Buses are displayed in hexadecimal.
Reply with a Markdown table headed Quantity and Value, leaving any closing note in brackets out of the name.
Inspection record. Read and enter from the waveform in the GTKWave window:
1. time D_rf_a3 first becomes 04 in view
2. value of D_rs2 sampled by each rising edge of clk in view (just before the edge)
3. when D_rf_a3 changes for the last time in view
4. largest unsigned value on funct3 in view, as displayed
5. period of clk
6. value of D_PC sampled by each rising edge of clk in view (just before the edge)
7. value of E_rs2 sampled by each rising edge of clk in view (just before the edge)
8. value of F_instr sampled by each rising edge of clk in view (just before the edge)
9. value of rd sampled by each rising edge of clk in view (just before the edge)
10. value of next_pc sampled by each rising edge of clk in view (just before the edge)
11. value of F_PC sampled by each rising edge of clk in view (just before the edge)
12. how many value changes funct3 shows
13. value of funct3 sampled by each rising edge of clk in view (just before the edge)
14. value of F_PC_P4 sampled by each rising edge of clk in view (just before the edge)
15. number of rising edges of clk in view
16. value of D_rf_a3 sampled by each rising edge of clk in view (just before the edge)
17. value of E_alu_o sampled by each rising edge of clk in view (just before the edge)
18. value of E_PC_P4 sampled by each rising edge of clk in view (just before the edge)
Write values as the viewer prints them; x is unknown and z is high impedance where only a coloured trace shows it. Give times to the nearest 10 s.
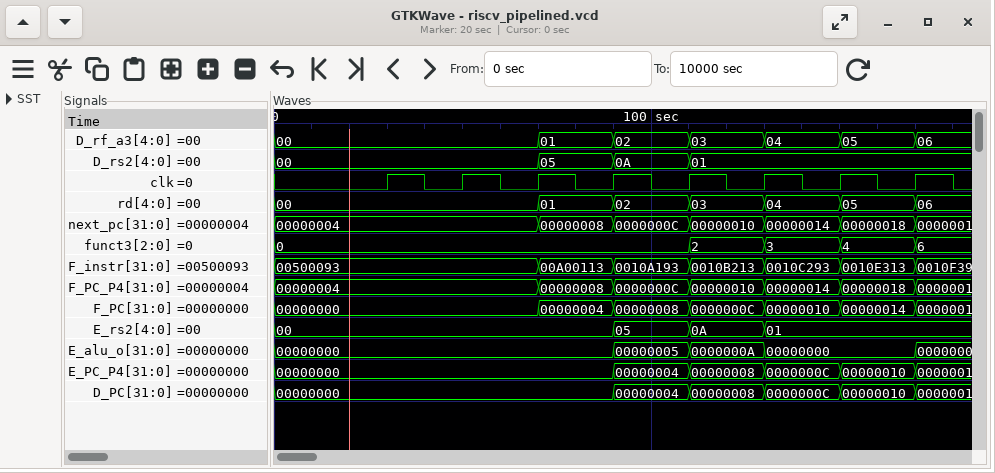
| Quantity | Value |
|---|---|
| time D_rf_a3 first becomes 04 in view | 130 s |
| value of D_rs2 sampled by each rising edge of clk in view | 00, 00, 00, 05, 0A, 01, 01, 01 |
| when D_rf_a3 changes for the last time in view | 170 s |
| largest unsigned value on funct3 in view, as displayed | 6 |
| period of clk | 20 s |
| value of D_PC sampled by each rising edge of clk in view | 00000000, 00000000, 00000000, 00000000, 00000004, 00000008, 0000000C, 00000010 |
| value of E_rs2 sampled by each rising edge of clk in view | 00, 00, 00, 00, 05, 0A, 01, 01 |
| value of F_instr sampled by each rising edge of clk in view | 00500093, 00500093, 00500093, 00A00113, 0010A193, 0010B213, 0010C293, 0010E313 |
| value of rd sampled by each rising edge of clk in view | 00, 00, 00, 01, 02, 03, 04, 05 |
| value of next_pc sampled by each rising edge of clk in view | 00000004, 00000004, 00000004, 00000008, 0000000C, 00000010, 00000014, 00000018 |
| value of F_PC sampled by each rising edge of clk in view | 00000000, 00000000, 00000000, 00000004, 00000008, 0000000C, 00000010, 00000014 |
| how many value changes funct3 shows | 4 |
| value of funct3 sampled by each rising edge of clk in view | 0, 0, 0, 0, 0, 2, 3, 4 |
| value of F_PC_P4 sampled by each rising edge of clk in view | 00000004, 00000004, 00000004, 00000008, 0000000C, 00000010, 00000014, 00000018 |
| number of rising edges of clk in view | 8 |
| value of D_rf_a3 sampled by each rising edge of clk in view | 00, 00, 00, 01, 02, 03, 04, 05 |
| value of E_alu_o sampled by each rising edge of clk in view | 00000000, 00000000, 00000000, 00000000, 00000005, 0000000A, 00000000, 00000000 |
| value of E_PC_P4 sampled by each rising edge of clk in view | 00000000, 00000000, 00000000, 00000000, 00000004, 00000008, 0000000C, 00000010 |
